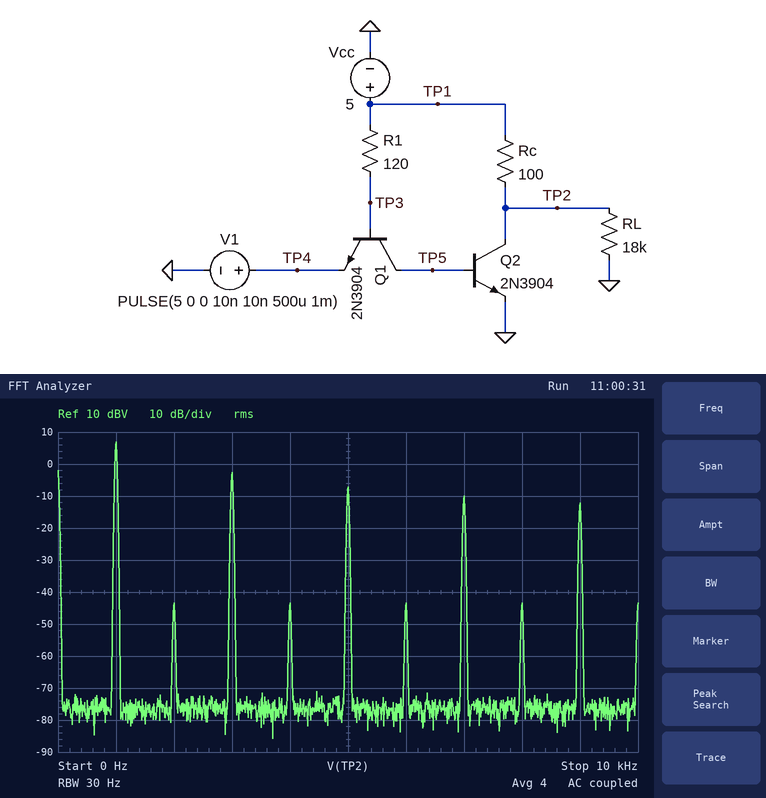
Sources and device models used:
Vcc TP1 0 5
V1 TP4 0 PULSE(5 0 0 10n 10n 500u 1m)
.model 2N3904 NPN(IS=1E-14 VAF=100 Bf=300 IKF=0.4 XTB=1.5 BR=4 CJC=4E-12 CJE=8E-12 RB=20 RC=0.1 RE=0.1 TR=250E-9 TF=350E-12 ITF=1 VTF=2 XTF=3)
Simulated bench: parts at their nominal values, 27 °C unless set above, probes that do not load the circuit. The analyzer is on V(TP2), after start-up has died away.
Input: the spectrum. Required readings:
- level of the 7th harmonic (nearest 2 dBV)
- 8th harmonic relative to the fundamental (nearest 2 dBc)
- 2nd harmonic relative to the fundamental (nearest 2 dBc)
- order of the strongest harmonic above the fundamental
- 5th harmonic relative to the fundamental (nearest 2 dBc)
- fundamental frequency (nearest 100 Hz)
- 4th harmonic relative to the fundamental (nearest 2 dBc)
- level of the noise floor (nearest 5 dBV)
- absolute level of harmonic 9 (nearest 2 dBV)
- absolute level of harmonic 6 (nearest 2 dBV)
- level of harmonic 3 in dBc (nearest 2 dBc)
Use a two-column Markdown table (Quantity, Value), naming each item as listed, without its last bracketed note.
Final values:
| Quantity | Value |
|---|---|
| level of the 7th harmonic | -10 dBV |
| 8th harmonic relative to the fundamental | -50 dBc |
| 2nd harmonic relative to the fundamental | -50 dBc |
| order of the strongest harmonic above the fundamental | 3 |
| 5th harmonic relative to the fundamental | -14 dBc |
| fundamental frequency | 1.0 kHz |
| 4th harmonic relative to the fundamental | -50 dBc |
| level of the noise floor | -75 dBV |
| absolute level of harmonic 9 | -12 dBV |
| absolute level of harmonic 6 | -44 dBV |
| level of harmonic 3 in dBc | -10 dBc |
